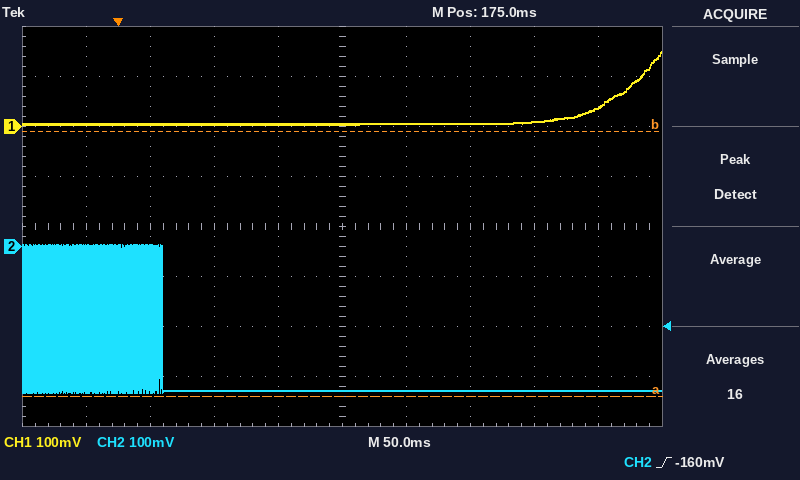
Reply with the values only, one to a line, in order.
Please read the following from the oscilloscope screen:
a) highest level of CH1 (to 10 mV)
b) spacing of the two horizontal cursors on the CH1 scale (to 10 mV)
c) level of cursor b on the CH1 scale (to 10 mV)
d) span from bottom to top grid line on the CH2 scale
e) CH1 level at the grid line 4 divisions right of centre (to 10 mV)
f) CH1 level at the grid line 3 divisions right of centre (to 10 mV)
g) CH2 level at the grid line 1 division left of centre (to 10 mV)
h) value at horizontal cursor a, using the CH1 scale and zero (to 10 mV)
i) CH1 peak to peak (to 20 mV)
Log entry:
150 mV
530 mV
-10 mV
800 mV
40 mV
10 mV
-290 mV
-540 mV
140 mV
